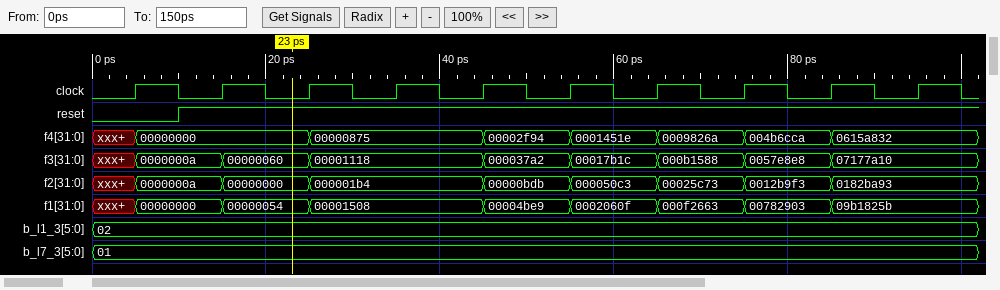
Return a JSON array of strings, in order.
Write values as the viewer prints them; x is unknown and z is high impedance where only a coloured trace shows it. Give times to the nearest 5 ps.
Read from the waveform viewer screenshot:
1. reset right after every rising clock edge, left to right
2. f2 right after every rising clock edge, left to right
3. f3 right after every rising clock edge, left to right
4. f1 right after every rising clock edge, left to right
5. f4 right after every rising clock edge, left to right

["0 1 1 1 1 1 1 1 1 1", "0000000a, 00000000, 000001b4, 000001b4, 00000bdb, 000050c3, 00025c73, 0012b9f3, 0182ba93, 0182ba93", "0000000a, 00000060, 00001118, 00001118, 000037a2, 00017b1c, 000b1588, 0057e8e8, 07177a10, 07177a10", "00000000, 00000054, 00001508, 00001508, 00004be9, 0002060f, 000f2663, 00782903, 09b1825b, 09b1825b", "00000000, 00000000, 00000875, 00000875, 00002f94, 0001451e, 0009826a, 004b6cca, 0615a832, 0615a832"]
